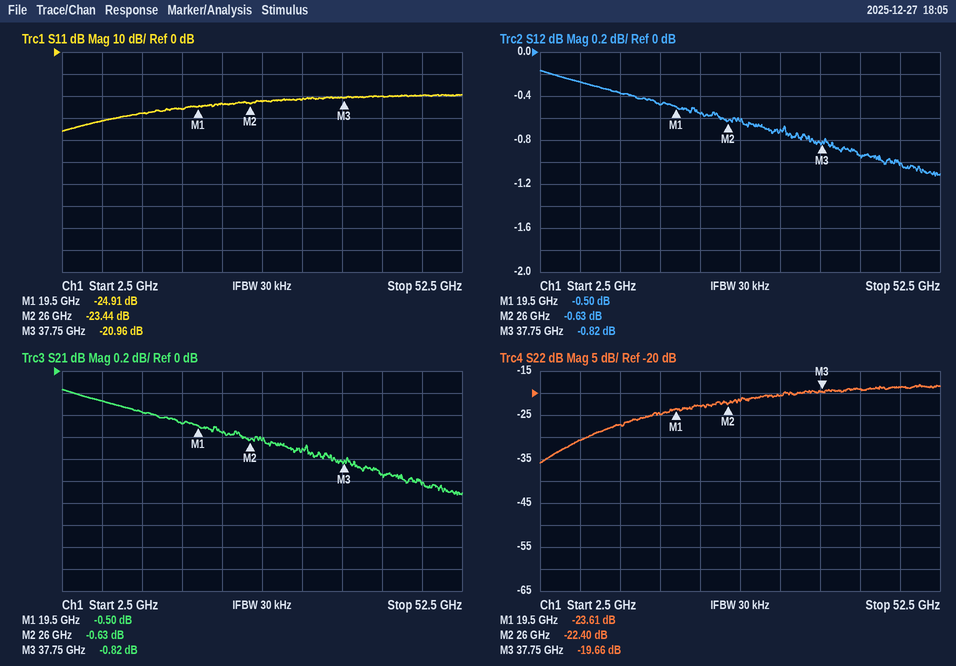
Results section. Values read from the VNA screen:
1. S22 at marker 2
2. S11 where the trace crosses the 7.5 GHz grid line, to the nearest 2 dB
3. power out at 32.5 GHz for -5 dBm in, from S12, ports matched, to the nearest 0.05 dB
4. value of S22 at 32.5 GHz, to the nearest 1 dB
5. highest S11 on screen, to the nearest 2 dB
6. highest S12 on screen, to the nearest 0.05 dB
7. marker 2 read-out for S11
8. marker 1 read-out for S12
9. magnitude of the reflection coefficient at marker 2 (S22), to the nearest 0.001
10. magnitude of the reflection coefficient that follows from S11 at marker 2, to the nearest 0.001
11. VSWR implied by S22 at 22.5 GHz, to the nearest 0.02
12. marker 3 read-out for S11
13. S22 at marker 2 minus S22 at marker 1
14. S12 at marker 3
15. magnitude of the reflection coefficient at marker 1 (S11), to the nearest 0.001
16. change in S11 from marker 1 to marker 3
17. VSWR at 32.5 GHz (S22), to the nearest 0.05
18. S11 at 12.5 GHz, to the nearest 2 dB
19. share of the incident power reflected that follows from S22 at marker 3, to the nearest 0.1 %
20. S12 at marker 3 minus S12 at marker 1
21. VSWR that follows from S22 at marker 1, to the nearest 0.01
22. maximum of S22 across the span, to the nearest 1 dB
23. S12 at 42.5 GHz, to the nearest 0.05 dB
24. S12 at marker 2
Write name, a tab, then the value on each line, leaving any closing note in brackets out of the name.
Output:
S22 at marker 2	-22.40 dB
S11 where the trace crosses the 7.5 GHz grid line, to the nearest 2 dB	-32 dB
power out at 32.5 GHz for -5 dBm in, from S12, ports matched, to the nearest 0.05 dB	-5.70 dBm
value of S22 at 32.5 GHz, to the nearest 1 dB	-21 dB
highest S11 on screen, to the nearest 2 dB	-20 dB
highest S12 on screen, to the nearest 0.05 dB	-0.15 dB
marker 2 read-out for S11	-23.44 dB
marker 1 read-out for S12	-0.50 dB
magnitude of the reflection coefficient at marker 2 (S22), to the nearest 0.001	0.076
magnitude of the reflection coefficient that follows from S11 at marker 2, to the nearest 0.001	0.067
VSWR implied by S22 at 22.5 GHz, to the nearest 0.02	1.16
marker 3 read-out for S11	-20.96 dB
S22 at marker 2 minus S22 at marker 1	1.21 dB
S12 at marker 3	-0.82 dB
magnitude of the reflection coefficient at marker 1 (S11), to the nearest 0.001	0.057
change in S11 from marker 1 to marker 3	3.95 dB
VSWR at 32.5 GHz (S22), to the nearest 0.05	1.20
S11 at 12.5 GHz, to the nearest 2 dB	-28 dB
share of the incident power reflected that follows from S22 at marker 3, to the nearest 0.1 %	1.1 %
S12 at marker 3 minus S12 at marker 1	-0.32 dB
VSWR that follows from S22 at marker 1, to the nearest 0.01	1.14
maximum of S22 across the span, to the nearest 1 dB	-18 dB
S12 at 42.5 GHz, to the nearest 0.05 dB	-0.95 dB
S12 at marker 2	-0.63 dB
